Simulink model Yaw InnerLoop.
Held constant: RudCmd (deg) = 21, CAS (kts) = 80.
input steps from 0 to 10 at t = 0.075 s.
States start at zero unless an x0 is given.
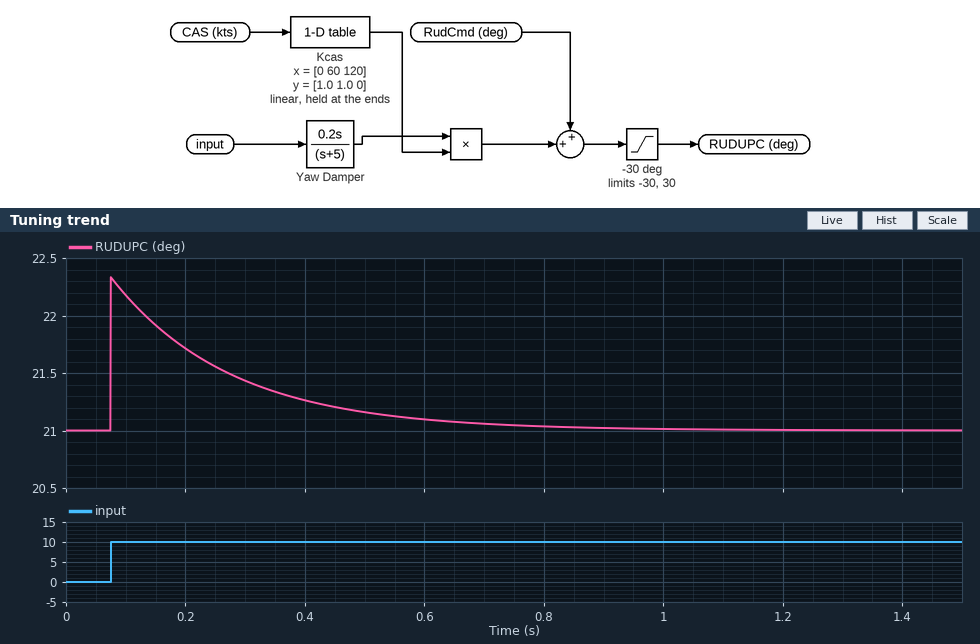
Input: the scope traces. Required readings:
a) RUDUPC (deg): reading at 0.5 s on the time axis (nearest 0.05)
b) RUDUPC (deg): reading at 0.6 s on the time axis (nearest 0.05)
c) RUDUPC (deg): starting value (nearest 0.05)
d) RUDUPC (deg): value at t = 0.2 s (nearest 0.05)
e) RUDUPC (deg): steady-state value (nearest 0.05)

21.15
21.10
21.00
21.70
21.00
